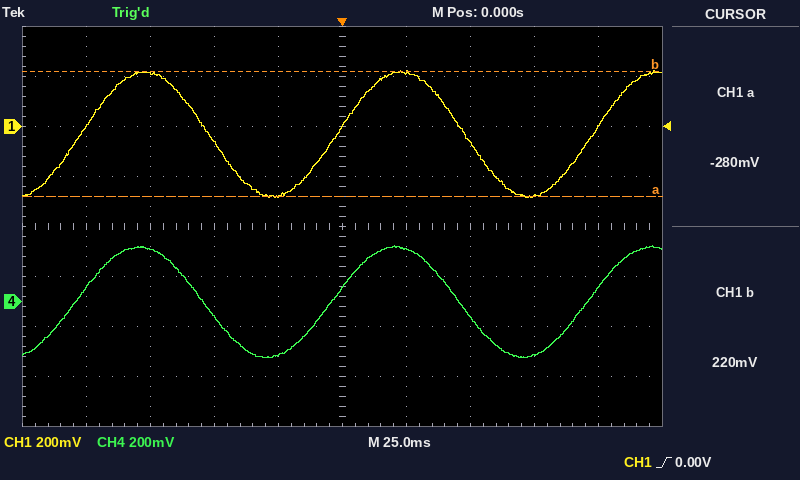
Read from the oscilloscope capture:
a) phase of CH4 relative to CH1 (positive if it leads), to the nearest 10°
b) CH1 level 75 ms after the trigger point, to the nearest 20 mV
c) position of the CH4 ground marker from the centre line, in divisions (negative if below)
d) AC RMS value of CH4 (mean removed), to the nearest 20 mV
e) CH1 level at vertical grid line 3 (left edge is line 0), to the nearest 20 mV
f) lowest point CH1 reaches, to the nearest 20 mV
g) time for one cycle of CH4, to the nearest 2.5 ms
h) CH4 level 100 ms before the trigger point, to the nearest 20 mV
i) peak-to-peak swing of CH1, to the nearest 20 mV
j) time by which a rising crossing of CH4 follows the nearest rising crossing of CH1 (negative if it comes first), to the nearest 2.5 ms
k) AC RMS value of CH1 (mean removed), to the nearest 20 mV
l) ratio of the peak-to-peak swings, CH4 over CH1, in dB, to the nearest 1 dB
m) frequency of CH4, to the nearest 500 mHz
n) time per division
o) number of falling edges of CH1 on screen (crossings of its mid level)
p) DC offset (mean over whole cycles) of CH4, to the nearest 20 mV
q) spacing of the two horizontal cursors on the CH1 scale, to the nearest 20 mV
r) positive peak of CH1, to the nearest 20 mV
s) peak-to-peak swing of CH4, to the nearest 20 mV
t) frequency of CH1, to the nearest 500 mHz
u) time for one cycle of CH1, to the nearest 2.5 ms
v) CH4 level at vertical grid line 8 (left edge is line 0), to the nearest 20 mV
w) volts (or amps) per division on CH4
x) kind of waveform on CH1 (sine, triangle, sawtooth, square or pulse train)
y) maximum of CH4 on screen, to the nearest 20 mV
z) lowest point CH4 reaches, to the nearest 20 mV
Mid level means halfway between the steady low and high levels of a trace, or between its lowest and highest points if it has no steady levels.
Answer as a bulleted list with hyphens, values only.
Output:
- +10°
- -280 mV
- -1.5 div
- 160 mV
- -60 mV
- -280 mV
- 100.0 ms
- 60 mV
- 500 mV
- -2.5 ms
- 180 mV
- -1 dB
- 10.0 Hz
- 25 ms
- 2
- 0 mV
- 500 mV
- 220 mV
- 440 mV
- 10.0 Hz
- 100.0 ms
- -220 mV
- 200 mV
- sine
- 220 mV
- -220 mV
